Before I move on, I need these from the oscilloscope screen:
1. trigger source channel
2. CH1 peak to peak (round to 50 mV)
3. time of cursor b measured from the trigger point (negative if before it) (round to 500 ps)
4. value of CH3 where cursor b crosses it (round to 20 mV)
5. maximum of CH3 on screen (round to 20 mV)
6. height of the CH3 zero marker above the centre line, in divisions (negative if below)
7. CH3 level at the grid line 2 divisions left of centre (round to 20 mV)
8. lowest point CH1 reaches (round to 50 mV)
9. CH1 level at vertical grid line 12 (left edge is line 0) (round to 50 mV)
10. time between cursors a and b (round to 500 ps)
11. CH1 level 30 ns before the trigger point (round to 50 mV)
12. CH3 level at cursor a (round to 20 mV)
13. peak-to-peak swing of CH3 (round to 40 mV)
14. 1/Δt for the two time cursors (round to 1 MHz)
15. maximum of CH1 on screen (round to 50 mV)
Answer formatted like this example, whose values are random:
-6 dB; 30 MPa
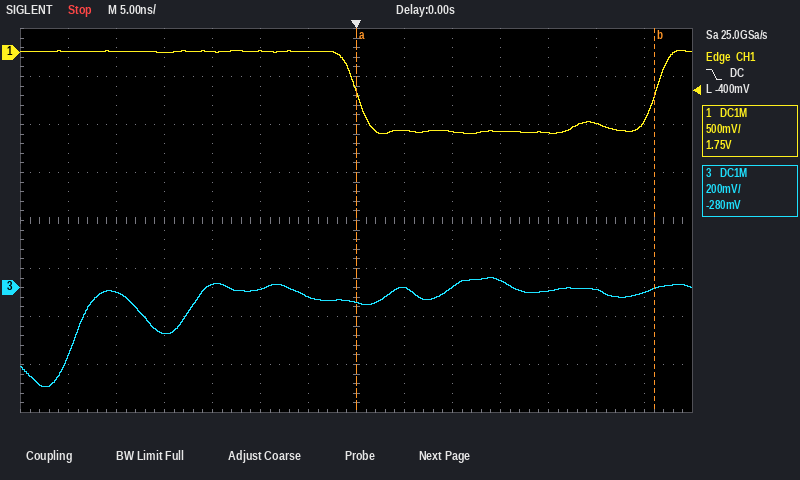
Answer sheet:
CH1; 850 mV; +31.0 ns; 0 mV; 40 mV; -1.4 div; 0 mV; -850 mV; -750 mV; 31.0 ns; 0 mV; -60 mV; 440 mV; 32 MHz; 0 mV
